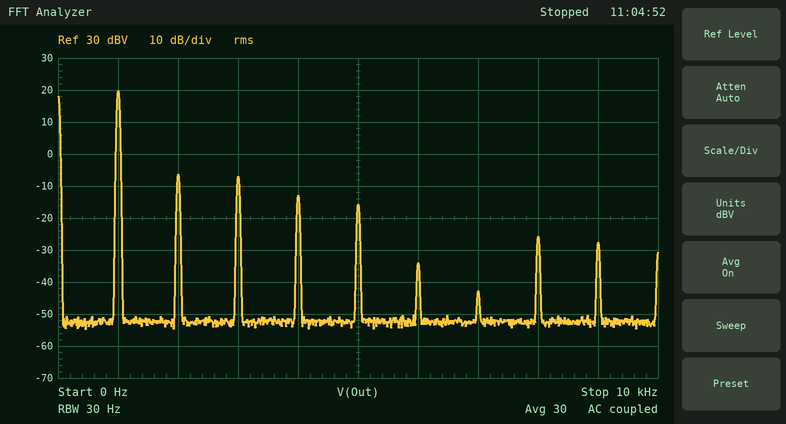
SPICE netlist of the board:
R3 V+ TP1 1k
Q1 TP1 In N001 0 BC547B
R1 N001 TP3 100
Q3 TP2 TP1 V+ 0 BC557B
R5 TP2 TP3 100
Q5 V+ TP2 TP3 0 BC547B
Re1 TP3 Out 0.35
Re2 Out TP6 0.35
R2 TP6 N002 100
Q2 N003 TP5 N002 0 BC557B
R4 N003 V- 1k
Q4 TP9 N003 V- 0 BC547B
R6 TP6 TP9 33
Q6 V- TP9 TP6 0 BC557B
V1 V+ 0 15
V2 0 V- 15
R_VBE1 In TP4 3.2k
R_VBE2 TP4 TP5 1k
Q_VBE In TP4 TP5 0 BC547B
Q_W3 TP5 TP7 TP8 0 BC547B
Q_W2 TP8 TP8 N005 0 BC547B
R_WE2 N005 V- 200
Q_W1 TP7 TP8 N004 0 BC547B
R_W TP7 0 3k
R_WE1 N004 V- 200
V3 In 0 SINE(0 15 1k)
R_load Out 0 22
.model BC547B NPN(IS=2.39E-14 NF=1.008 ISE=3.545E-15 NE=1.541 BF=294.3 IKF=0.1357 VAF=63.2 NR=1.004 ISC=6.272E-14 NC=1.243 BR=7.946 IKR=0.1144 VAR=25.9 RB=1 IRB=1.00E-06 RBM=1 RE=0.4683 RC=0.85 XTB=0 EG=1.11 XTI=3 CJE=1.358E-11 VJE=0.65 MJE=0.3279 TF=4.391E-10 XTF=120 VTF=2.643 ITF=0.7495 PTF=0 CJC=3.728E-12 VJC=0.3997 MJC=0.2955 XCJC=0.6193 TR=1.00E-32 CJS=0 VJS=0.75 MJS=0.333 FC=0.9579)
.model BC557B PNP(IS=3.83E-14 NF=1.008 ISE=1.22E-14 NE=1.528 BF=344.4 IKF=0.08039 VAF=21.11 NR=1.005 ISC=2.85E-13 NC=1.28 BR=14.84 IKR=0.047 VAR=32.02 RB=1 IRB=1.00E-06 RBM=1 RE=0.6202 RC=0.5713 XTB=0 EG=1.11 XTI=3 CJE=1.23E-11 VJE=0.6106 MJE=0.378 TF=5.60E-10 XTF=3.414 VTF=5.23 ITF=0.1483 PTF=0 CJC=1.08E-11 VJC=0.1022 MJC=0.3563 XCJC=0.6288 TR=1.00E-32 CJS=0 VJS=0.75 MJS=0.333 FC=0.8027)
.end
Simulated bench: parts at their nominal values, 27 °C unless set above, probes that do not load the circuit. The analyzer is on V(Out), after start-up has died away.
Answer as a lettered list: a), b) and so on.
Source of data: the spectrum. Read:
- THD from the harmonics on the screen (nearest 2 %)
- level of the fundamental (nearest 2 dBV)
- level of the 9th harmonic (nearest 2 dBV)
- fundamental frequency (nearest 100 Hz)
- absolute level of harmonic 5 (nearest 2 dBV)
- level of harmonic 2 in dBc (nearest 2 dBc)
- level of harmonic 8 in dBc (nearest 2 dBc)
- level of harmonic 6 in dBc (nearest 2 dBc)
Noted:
a) 8 %
b) 20 dBV
c) -28 dBV
d) 1.0 kHz
e) -16 dBV
f) -26 dBc
g) -46 dBc
h) -54 dBc
